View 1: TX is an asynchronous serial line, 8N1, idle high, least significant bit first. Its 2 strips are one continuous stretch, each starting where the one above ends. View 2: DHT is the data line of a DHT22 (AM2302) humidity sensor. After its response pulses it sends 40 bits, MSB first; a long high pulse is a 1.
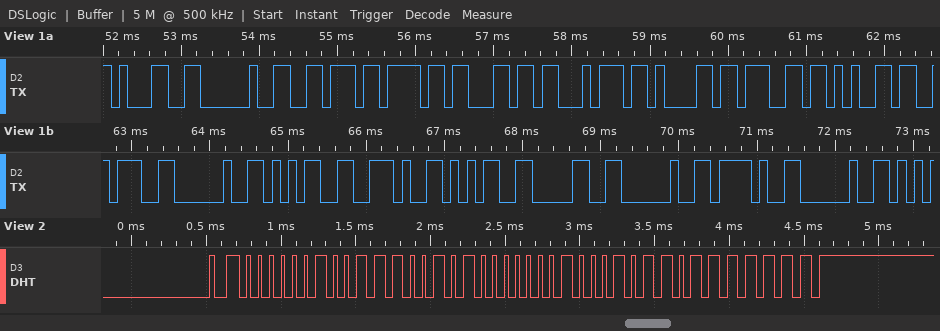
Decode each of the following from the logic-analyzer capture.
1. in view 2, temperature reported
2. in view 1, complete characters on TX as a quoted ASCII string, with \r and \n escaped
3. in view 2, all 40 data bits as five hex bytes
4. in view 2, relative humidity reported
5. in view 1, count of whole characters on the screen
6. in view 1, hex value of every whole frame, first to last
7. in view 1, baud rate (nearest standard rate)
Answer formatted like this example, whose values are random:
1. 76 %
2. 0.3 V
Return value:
1. -13.9 °C
2. "1 voltage: 5.50 / "
3. 02 72 80 8B 7F
4. 62.6 %
5. 18
6. 31 20 76 6F 6C 74 61 67 65 3A 20 35 2E 35 30 20 2F 20
7. 9600 baud
